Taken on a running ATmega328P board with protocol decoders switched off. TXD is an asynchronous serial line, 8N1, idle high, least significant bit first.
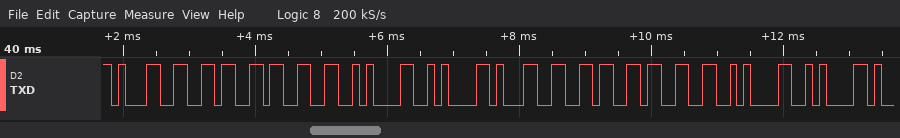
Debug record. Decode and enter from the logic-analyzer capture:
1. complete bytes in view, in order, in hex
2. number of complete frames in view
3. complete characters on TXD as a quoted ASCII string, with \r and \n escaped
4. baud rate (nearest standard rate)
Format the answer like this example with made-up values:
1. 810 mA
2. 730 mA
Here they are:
1. 0x31 0x36 0x33 0x0A 0x0A 0x31 0x36 0x33 0x0A 0x0A
2. 10
3. "163\n\n163\n\n"
4. 9600 baud
